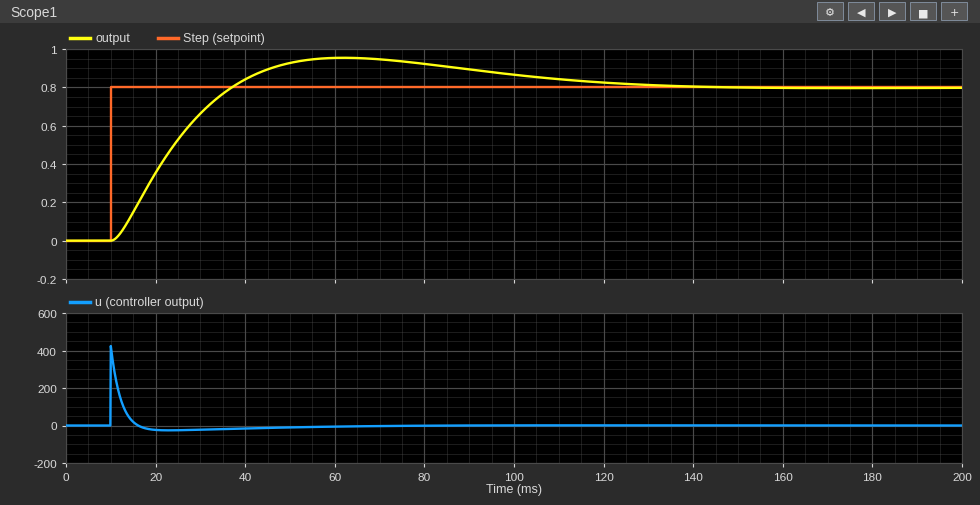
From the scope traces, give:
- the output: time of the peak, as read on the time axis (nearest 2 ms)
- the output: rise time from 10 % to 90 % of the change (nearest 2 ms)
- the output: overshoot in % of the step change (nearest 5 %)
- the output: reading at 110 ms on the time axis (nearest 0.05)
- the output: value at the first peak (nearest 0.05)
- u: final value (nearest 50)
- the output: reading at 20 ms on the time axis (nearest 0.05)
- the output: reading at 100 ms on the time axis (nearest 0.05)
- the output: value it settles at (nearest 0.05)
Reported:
62 ms
20 ms
20 %
0.85
0.95
0
0.35
0.85
0.80
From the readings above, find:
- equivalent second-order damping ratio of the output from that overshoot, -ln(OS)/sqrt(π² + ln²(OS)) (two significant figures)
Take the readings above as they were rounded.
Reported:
0.46
